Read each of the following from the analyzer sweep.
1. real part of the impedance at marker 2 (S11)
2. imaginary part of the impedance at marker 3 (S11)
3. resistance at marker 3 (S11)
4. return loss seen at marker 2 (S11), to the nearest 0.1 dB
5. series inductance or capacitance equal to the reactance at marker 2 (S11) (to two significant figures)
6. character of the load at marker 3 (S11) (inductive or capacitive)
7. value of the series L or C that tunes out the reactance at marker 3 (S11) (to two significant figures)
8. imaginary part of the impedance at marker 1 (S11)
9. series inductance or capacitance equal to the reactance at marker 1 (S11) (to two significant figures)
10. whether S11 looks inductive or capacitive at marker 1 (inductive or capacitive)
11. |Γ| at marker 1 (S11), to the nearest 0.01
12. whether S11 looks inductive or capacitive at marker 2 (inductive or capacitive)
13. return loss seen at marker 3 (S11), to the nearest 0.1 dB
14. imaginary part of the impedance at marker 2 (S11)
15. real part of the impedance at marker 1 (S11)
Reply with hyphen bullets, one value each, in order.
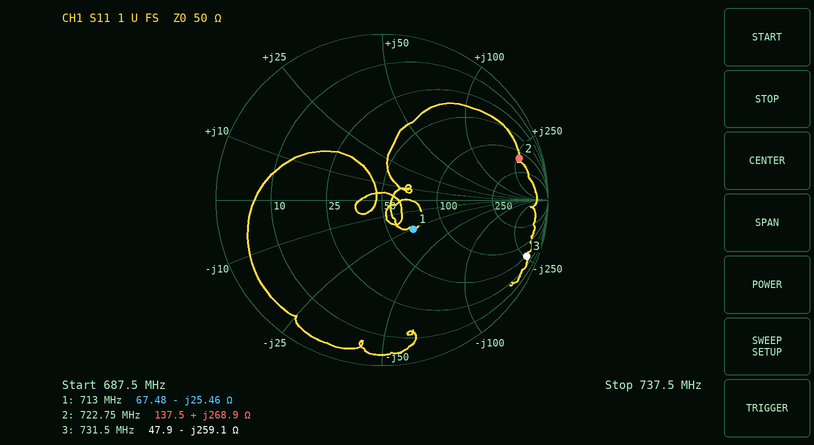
- 137.5 Ω
- -259.1 Ω
- 47.9 Ω
- 1.3 dB
- 59 nH
- capacitive
- 56 nH
- -25.46 Ω
- 8.8 pF
- capacitive
- 0.26
- inductive
- 0.6 dB
- +268.9 Ω
- 67.48 Ω
